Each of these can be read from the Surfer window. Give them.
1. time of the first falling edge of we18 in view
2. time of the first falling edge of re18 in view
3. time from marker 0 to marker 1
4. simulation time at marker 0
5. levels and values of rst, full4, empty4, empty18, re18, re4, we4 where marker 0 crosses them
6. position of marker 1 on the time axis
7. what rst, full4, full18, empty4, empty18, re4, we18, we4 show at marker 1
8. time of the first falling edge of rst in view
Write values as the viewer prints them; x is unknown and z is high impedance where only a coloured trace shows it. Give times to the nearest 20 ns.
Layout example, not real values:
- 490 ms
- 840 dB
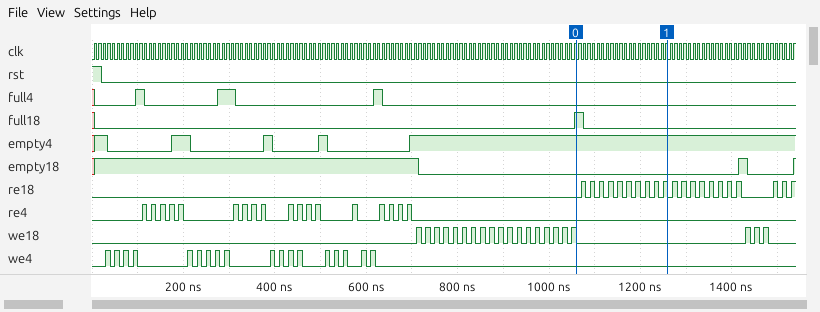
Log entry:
- 720 ns
- 1080 ns
- 200 ns
- 1060 ns
- rst=0, full4=0, empty4=1, empty18=0, re18=0, re4=0, we4=0
- 1260 ns
- rst=0, full4=0, full18=0, empty4=1, empty18=0, re4=0, we18=0, we4=0
- 20 ns
